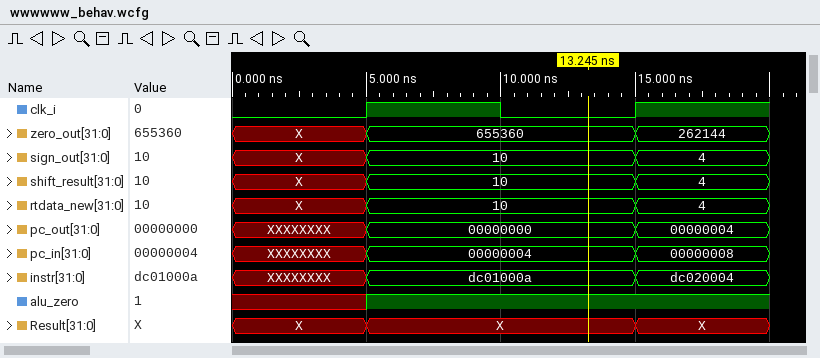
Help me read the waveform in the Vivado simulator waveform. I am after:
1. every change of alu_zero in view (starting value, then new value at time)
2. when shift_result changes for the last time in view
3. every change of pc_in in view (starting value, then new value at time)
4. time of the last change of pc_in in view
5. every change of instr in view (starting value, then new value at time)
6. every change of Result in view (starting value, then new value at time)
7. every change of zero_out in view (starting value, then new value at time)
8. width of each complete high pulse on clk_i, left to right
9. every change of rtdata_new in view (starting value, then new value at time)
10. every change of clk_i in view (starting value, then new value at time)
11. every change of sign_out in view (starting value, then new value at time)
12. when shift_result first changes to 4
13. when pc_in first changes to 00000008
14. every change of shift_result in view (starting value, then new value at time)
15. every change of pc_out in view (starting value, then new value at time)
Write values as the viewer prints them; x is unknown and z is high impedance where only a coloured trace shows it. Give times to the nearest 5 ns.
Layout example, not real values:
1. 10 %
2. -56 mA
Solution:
1. x, 1 at 5 ns
2. 15 ns
3. XXXXXXXX, 00000004 at 5 ns, 00000008 at 15 ns
4. 15 ns
5. XXXXXXXX, dc01000a at 5 ns, dc020004 at 15 ns
6. X, X at 5 ns, X at 15 ns
7. X, 655360 at 5 ns, 262144 at 15 ns
8. 5 ns
9. X, 10 at 5 ns, 4 at 15 ns
10. 0, 1 at 5 ns, 0 at 10 ns, 1 at 15 ns
11. X, 10 at 5 ns, 4 at 15 ns
12. 15 ns
13. 15 ns
14. X, 10 at 5 ns, 4 at 15 ns
15. XXXXXXXX, 00000000 at 5 ns, 00000004 at 15 ns
